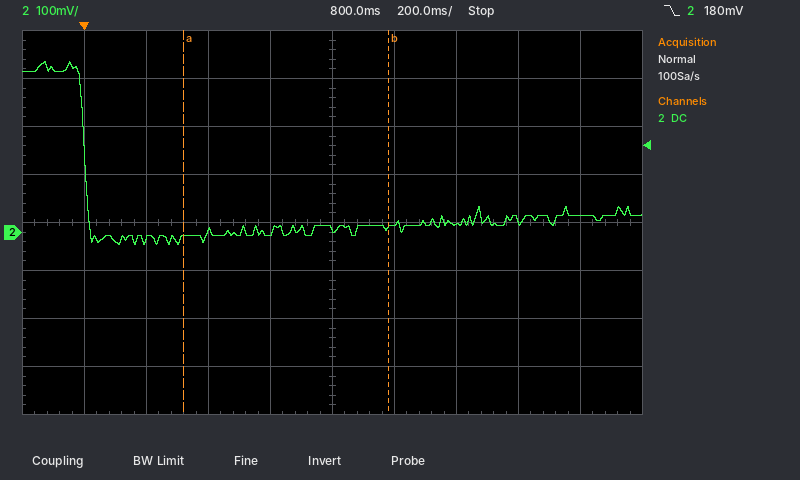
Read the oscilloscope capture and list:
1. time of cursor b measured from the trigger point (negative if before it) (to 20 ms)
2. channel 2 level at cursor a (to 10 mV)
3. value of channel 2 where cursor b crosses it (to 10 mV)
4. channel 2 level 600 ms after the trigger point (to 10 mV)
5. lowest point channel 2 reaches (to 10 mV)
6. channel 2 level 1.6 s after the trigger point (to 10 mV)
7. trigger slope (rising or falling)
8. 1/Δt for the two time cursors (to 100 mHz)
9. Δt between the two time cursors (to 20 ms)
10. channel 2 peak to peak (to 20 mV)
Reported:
+980 ms
-10 mV
10 mV
0 mV
-30 mV
30 mV
falling
1.5 Hz
660 ms
380 mV
